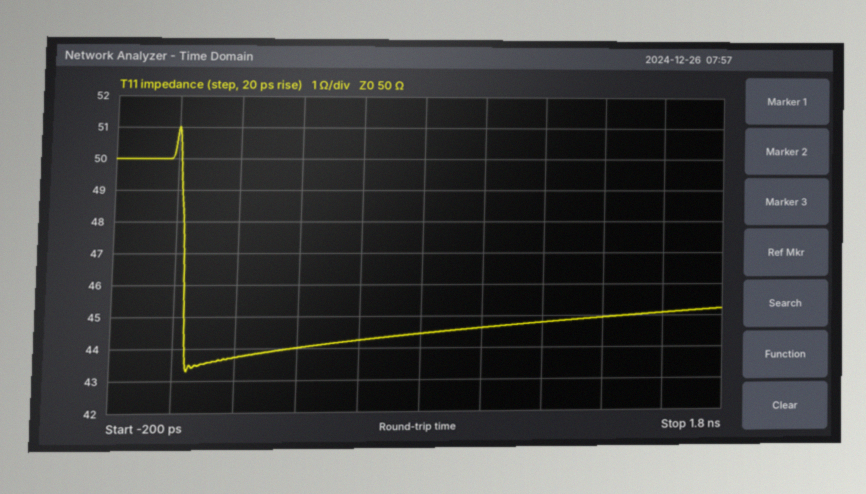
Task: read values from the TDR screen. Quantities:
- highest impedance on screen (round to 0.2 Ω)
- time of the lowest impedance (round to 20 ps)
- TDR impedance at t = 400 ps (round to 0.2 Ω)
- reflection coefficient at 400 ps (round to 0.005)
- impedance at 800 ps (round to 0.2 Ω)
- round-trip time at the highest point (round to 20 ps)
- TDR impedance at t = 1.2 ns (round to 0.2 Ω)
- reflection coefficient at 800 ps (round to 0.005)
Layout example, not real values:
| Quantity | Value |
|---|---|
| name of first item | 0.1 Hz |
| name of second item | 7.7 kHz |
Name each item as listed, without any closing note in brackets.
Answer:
| Quantity | Value |
|---|---|
| highest impedance on screen | 51.0 Ω |
| time of the lowest impedance | 40 ps |
| TDR impedance at t = 400 ps | 44.0 Ω |
| reflection coefficient at 400 ps | -0.065 |
| impedance at 800 ps | 44.4 Ω |
| round-trip time at the highest point | 0 ps |
| TDR impedance at t = 1.2 ns | 44.8 Ω |
| reflection coefficient at 800 ps | -0.060 |
